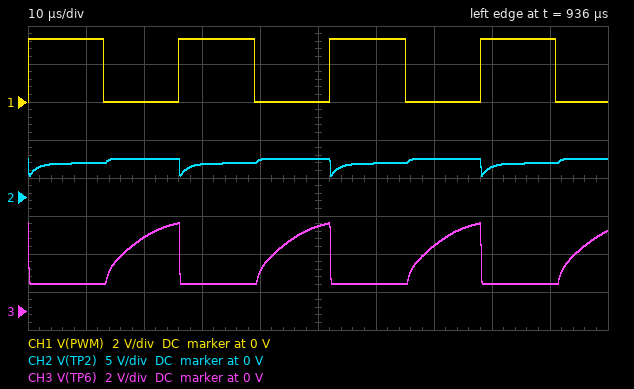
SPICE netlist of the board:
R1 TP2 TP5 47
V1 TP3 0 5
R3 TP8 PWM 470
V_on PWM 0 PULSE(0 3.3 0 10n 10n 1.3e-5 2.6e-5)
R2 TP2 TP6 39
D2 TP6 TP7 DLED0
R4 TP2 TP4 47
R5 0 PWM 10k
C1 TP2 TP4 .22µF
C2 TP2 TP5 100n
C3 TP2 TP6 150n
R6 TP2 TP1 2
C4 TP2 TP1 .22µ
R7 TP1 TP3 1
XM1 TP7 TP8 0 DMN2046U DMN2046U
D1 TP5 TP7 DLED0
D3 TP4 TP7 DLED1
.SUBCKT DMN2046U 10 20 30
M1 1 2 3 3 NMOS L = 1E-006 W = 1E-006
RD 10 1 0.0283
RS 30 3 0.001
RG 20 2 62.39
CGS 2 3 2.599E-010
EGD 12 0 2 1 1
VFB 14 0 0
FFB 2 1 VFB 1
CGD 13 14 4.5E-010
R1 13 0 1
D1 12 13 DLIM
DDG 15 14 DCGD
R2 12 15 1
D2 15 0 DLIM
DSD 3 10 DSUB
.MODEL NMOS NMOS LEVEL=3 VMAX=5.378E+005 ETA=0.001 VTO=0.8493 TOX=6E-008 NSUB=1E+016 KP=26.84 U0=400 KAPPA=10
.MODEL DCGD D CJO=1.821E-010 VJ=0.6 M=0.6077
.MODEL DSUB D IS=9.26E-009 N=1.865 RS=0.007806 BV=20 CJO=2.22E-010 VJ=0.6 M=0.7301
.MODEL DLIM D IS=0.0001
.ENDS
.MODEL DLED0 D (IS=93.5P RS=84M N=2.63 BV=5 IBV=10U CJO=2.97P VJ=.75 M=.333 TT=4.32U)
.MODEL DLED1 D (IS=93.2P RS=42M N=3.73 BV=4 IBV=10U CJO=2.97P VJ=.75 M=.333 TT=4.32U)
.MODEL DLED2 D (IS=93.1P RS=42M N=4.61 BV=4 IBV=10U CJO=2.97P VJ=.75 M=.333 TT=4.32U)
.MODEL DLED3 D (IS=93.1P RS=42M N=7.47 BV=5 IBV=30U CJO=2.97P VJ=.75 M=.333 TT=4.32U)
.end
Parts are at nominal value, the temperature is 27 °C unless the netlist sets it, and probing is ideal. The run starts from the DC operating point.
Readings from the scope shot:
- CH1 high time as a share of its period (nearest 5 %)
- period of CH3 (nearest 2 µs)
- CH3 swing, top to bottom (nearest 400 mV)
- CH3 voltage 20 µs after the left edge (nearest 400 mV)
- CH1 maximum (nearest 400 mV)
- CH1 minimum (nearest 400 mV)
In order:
50 %
26 µs
3.2 V
4.0 V
3.2 V
0 V
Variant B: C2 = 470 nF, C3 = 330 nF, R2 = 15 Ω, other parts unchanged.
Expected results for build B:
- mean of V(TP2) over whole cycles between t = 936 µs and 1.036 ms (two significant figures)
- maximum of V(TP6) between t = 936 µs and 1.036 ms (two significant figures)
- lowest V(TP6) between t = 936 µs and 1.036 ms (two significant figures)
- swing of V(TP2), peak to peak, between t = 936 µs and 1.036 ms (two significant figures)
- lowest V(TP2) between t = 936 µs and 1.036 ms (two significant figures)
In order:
4.4 V
4.7 V
1.5 V
2.4 V
2.6 V
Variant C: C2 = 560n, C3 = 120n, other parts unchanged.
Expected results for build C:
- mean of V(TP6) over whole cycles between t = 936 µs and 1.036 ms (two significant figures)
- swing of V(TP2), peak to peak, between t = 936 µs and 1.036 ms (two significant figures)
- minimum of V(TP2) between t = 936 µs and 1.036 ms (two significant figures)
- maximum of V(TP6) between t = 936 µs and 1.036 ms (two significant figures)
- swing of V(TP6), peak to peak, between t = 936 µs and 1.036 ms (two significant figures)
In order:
2.3 V
2.0 V
3.0 V
4.5 V
3.1 V
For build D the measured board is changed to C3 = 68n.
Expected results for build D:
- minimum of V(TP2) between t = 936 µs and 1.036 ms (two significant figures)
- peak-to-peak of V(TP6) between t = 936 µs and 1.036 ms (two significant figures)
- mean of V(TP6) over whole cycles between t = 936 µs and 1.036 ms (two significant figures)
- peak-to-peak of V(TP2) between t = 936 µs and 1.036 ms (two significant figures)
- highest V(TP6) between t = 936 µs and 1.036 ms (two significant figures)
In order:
2.8 V
3.5 V
2.6 V
2.2 V
4.9 V
